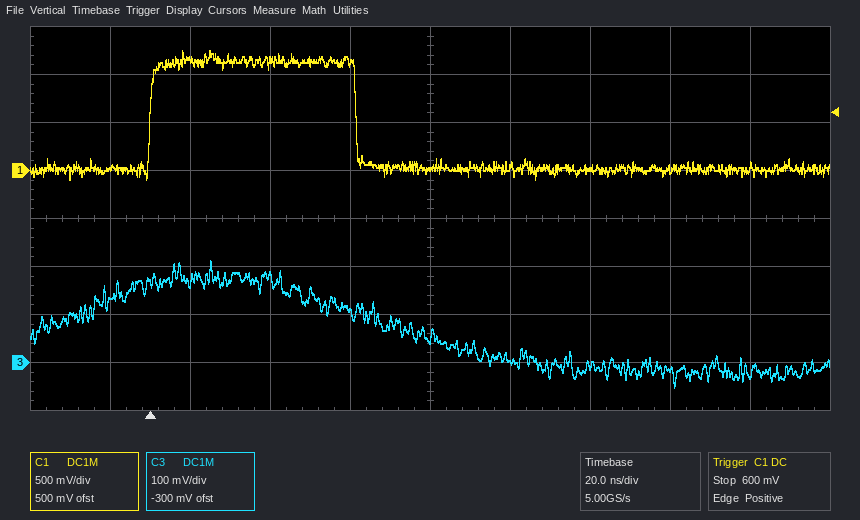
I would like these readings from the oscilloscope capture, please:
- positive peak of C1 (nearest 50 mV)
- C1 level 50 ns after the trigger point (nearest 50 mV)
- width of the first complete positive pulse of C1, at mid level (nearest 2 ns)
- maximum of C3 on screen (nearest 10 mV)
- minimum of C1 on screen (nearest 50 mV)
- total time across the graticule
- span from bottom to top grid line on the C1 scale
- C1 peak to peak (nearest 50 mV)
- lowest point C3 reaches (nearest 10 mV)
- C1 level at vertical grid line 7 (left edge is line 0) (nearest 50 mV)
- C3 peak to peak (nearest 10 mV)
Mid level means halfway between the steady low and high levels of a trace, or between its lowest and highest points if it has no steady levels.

1.25 V
1.15 V
52 ns
210 mV
-100 mV
200 ns
4 V
1.35 V
-50 mV
0 mV
260 mV
